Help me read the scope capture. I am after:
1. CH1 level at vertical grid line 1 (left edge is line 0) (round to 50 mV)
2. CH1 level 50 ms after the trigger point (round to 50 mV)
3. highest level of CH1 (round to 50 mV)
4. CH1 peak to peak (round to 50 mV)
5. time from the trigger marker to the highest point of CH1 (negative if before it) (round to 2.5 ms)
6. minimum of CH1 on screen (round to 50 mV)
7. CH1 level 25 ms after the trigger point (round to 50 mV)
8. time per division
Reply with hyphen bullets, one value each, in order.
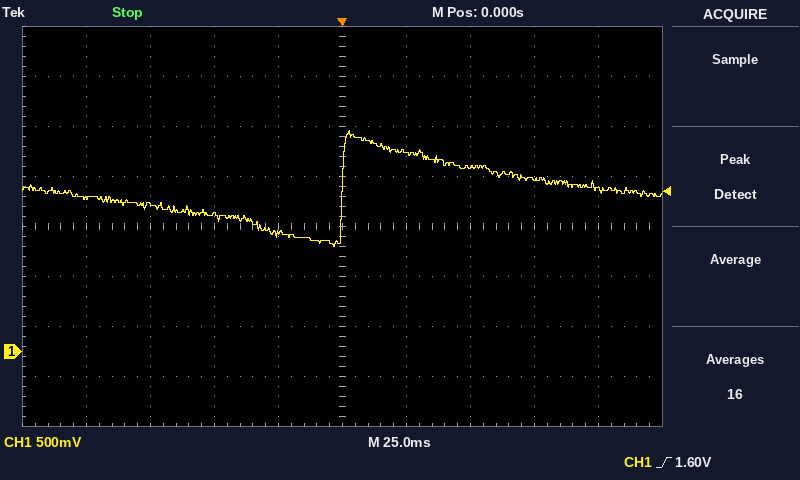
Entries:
- 1.55 V
- 1.85 V
- 2.20 V
- 1.15 V
- +2.5 ms
- 1.05 V
- 2.00 V
- 25 ms
